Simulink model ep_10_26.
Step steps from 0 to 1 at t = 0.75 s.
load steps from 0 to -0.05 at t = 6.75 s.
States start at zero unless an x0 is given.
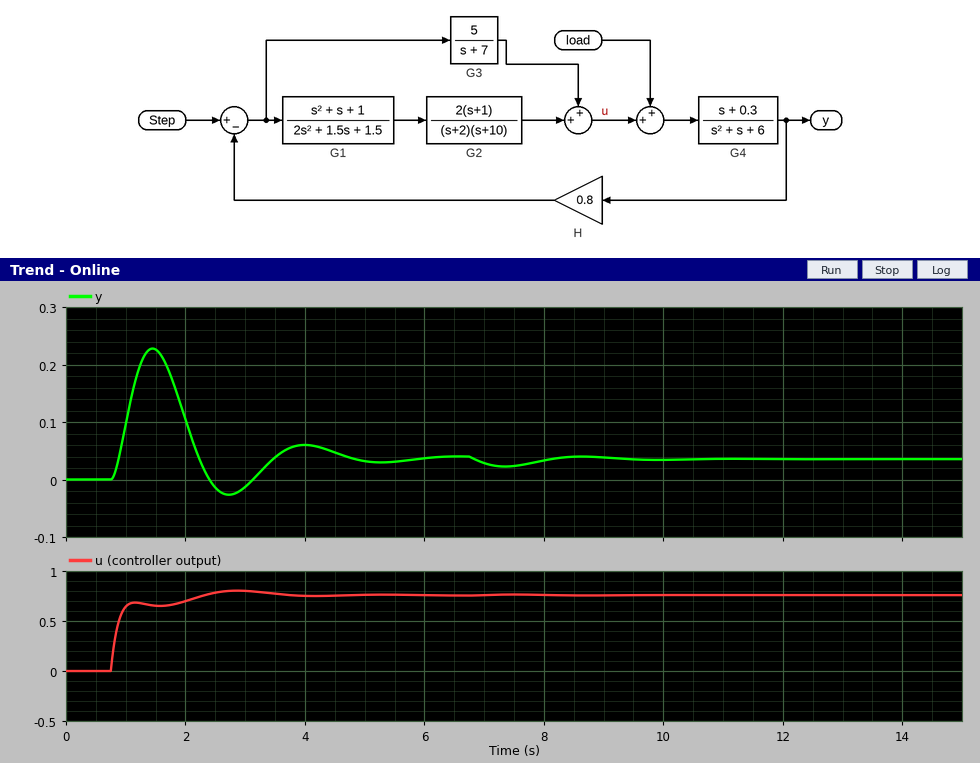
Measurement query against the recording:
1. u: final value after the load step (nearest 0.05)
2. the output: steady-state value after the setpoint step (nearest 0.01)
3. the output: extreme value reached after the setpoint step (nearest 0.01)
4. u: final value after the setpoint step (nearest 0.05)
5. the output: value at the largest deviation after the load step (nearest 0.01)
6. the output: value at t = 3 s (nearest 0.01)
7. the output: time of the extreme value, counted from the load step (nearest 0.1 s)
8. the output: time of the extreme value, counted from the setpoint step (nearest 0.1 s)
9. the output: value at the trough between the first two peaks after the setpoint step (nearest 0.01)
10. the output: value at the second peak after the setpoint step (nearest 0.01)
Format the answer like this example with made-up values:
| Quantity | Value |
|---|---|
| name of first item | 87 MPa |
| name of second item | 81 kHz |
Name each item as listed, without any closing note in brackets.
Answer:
| Quantity | Value |
|---|---|
| u: final value after the load step | 0.75 |
| the output: steady-state value after the setpoint step | 0.04 |
| the output: extreme value reached after the setpoint step | 0.23 |
| u: final value after the setpoint step | 0.75 |
| the output: value at the largest deviation after the load step | 0.02 |
| the output: value at t = 3 s | -0.01 |
| the output: time of the extreme value, counted from the load step | 0.6 s |
| the output: time of the extreme value, counted from the setpoint step | 0.7 s |
| the output: value at the trough between the first two peaks after the setpoint step | -0.03 |
| the output: value at the second peak after the setpoint step | 0.06 |
